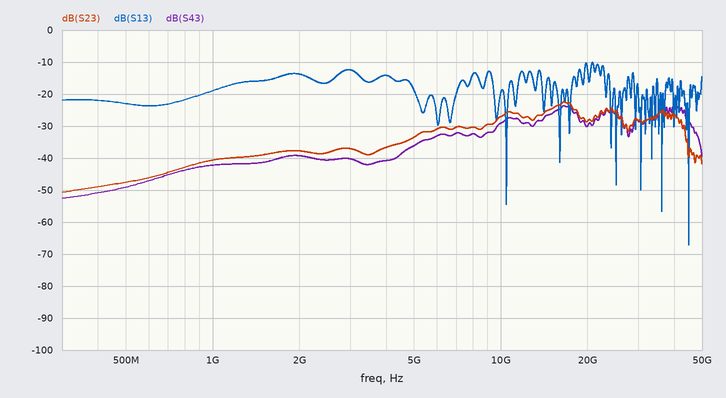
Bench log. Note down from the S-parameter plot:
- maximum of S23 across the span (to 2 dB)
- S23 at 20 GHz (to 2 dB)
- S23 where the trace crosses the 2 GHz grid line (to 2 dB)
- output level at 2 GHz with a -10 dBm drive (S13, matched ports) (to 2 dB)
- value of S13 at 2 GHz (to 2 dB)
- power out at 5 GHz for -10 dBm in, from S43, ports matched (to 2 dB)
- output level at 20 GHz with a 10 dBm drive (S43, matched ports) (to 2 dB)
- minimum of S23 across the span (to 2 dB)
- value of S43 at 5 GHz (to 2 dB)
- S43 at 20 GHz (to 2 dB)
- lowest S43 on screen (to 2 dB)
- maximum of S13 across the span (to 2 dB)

-22 dB
-28 dB
-38 dB
-24 dBm
-14 dB
-46 dBm
-20 dBm
-50 dB
-36 dB
-30 dB
-52 dB
-10 dB
